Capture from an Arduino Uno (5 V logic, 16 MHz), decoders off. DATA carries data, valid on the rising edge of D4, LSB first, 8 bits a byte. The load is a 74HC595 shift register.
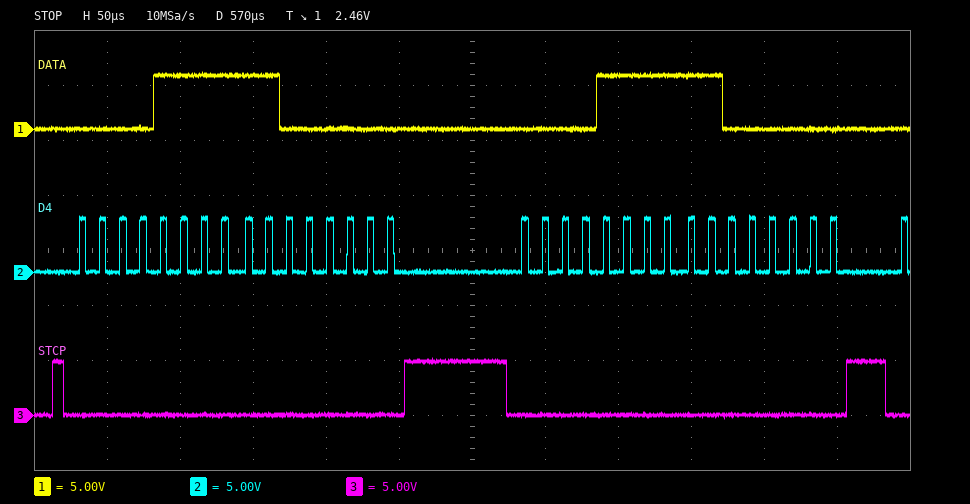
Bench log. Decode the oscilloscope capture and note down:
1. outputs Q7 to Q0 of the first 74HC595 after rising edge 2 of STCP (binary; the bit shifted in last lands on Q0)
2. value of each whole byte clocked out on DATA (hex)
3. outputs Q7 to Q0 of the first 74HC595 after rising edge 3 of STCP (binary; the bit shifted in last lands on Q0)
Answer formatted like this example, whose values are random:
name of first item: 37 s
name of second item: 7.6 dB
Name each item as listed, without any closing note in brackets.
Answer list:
outputs Q7 to Q0 of the first 74HC595 after rising edge 2 of STCP: 11000000
value of each whole byte clocked out on DATA: F0 03 F0 03
outputs Q7 to Q0 of the first 74HC595 after rising edge 3 of STCP: 11000000
